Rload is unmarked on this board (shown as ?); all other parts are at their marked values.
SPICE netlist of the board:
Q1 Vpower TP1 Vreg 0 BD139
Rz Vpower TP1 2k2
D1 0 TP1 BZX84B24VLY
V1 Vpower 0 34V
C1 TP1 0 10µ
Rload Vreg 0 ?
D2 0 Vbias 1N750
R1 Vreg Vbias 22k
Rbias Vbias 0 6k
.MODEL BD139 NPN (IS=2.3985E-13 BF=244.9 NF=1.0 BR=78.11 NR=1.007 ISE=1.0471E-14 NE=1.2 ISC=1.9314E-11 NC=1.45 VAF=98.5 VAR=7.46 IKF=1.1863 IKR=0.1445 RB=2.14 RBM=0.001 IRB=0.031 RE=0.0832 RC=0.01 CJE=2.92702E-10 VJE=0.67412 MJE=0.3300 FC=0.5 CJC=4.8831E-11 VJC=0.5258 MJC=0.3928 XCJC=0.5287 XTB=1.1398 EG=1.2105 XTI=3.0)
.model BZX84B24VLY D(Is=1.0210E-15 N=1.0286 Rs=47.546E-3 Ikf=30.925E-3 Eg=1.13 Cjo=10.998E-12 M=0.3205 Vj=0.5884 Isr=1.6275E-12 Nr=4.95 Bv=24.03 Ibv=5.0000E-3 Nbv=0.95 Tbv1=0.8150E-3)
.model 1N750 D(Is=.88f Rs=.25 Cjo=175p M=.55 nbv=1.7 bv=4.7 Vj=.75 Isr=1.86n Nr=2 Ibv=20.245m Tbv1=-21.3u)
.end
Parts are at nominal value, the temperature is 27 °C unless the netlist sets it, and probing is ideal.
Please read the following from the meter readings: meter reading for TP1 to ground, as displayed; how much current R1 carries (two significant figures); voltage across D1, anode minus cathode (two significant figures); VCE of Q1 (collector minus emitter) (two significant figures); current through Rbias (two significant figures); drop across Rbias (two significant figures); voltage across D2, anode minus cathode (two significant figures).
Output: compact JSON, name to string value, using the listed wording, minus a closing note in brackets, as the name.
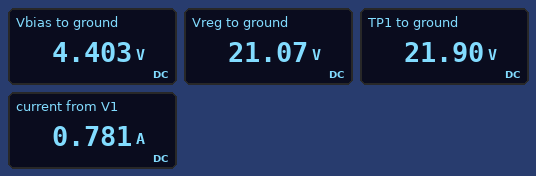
{"meter reading for TP1 to ground, as displayed": "21.90 V", "how much current R1 carries": "760 µA", "voltage across D1, anode minus cathode": "-22 V", "VCE of Q1 (collector minus emitter)": "13 V", "current through Rbias": "730 µA", "drop across Rbias": "4.4 V", "voltage across D2, anode minus cathode": "-4.4 V"}
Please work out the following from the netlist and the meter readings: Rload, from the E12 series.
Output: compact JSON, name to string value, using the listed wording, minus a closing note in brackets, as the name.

{"Rload, from the E12 series": "27 Ω"}
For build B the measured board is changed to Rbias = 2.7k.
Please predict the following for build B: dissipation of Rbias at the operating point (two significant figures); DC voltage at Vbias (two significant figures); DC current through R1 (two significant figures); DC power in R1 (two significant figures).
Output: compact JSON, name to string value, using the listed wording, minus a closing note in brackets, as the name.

{"dissipation of Rbias at the operating point": "2.0 mW", "DC voltage at Vbias": "2.3 V", "DC current through R1": "850 µA", "DC power in R1": "16 mW"}
